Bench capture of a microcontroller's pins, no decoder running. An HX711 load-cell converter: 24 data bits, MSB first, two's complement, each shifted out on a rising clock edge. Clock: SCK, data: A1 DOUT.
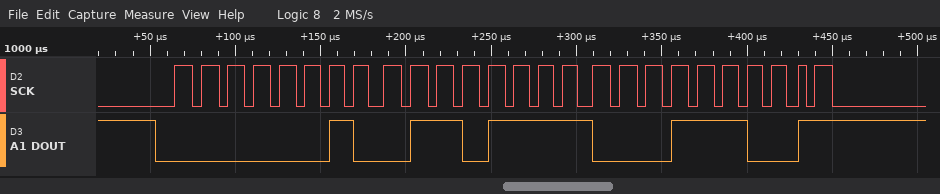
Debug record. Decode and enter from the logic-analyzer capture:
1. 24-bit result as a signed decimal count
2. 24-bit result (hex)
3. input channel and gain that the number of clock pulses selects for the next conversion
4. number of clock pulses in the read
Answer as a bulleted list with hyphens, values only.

- 159516
- 0x026F1C
- channel B, gain 32
- 26
